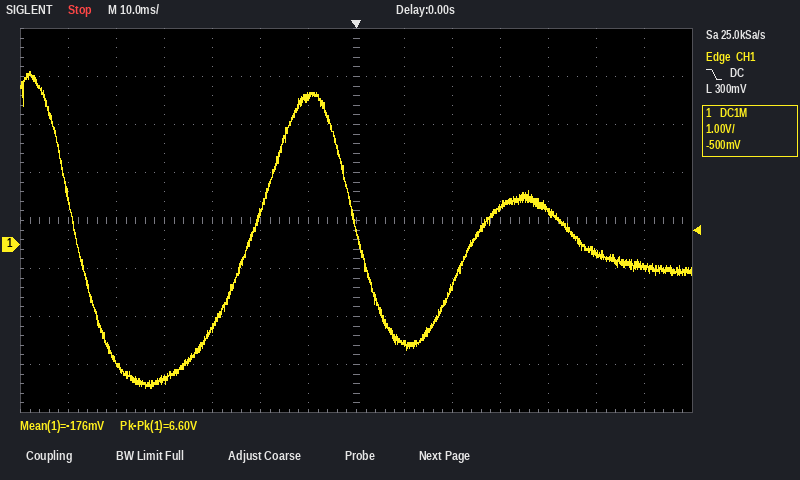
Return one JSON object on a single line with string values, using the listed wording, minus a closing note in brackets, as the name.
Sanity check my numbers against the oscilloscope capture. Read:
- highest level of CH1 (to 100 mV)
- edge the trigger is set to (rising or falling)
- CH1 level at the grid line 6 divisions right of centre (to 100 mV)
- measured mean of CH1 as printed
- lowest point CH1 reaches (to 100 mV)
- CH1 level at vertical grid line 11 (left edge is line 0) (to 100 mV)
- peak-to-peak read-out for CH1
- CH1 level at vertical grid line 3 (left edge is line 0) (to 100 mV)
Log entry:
{"highest level of CH1": "3.6 V", "edge the trigger is set to": "falling", "CH1 level at the grid line 6 divisions right of centre": "-500 mV", "measured mean of CH1 as printed": "-176 mV", "lowest point CH1 reaches": "-3.0 V", "CH1 level at vertical grid line 11 (left edge is line 0)": "700 mV", "peak-to-peak read-out for CH1": "6.60 V", "CH1 level at vertical grid line 3 (left edge is line 0)": "-2.8 V"}
